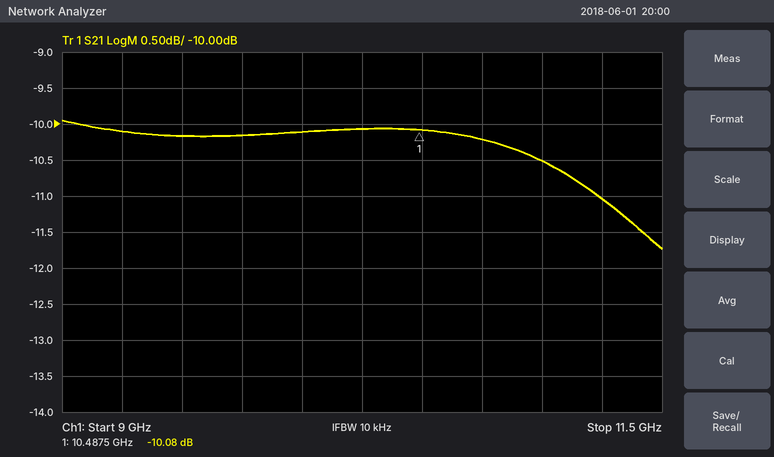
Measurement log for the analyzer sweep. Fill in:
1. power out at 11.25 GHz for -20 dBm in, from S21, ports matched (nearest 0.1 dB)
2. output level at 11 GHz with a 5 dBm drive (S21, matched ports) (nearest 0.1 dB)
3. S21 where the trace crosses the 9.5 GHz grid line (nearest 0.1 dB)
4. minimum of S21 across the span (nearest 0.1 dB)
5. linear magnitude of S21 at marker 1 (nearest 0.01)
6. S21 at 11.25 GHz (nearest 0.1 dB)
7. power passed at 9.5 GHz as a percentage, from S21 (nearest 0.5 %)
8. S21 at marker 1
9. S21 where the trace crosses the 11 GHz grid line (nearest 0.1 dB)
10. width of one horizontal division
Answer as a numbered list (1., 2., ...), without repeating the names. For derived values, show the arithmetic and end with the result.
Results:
1. -20 dBm + (-11.0 dB) = -31.0 dBm
2. 5 dBm + (-10.5 dB) = -5.5 dBm
3. -10.2 dB
4. -11.7 dB
5. 10^(-10.08/20) ≈ 0.31
6. -11.0 dB
7. 10^(-10.2/10) ≈ 9.5 %
8. -10.08 dB
9. -10.5 dB
10. 250 MHz
